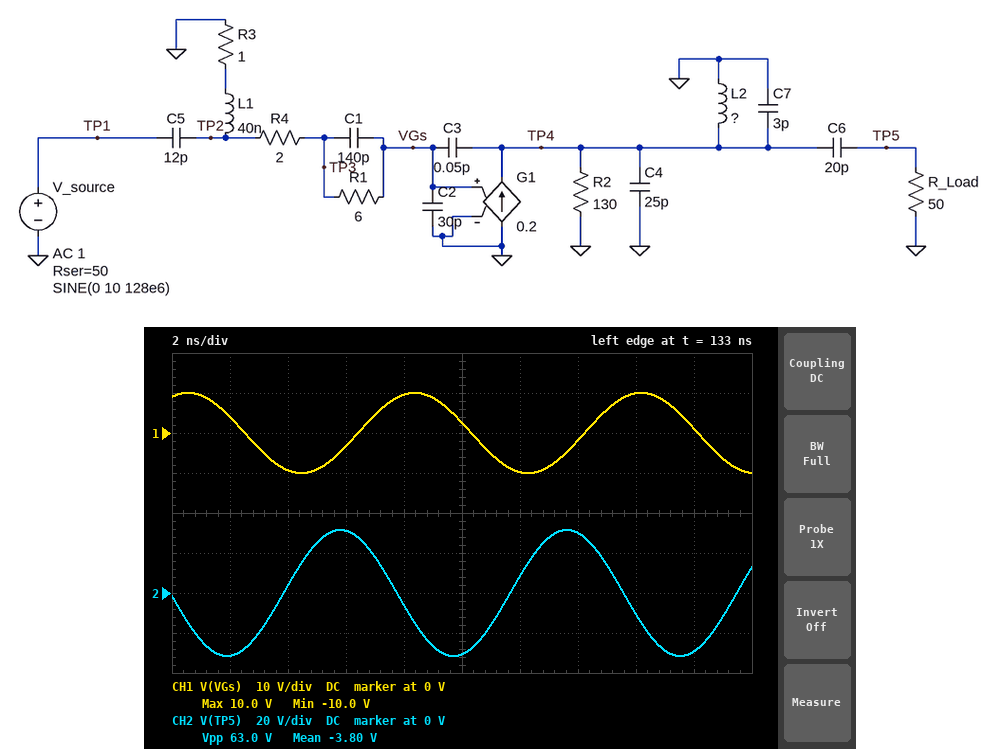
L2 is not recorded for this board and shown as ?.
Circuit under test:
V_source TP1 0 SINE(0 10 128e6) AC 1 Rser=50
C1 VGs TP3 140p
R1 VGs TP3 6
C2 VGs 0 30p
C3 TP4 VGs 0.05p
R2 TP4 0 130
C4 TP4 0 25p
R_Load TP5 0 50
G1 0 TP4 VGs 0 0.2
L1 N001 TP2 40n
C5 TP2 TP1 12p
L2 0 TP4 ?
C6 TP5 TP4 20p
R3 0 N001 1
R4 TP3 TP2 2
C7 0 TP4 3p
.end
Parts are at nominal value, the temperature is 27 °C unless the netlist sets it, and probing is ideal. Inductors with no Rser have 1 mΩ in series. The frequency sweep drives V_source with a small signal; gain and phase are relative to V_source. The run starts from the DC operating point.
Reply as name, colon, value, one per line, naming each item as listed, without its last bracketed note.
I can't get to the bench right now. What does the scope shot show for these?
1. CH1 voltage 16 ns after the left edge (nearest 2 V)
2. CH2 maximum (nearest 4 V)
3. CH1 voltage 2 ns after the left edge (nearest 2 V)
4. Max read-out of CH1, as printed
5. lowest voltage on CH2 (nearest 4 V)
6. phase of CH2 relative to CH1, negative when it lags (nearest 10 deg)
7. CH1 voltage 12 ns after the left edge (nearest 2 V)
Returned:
CH1 voltage 16 ns after the left edge: 10 V
CH2 maximum: 32 V
CH1 voltage 2 ns after the left edge: 4 V
Max read-out of CH1, as printed: 10.0 V
lowest voltage on CH2: -32 V
phase of CH2 relative to CH1, negative when it lags: 120 deg
CH1 voltage 12 ns after the left edge: -10 V
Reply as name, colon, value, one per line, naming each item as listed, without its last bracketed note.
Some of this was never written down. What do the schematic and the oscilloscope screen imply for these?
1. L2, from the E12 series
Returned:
L2, from the E12 series: 18 nH
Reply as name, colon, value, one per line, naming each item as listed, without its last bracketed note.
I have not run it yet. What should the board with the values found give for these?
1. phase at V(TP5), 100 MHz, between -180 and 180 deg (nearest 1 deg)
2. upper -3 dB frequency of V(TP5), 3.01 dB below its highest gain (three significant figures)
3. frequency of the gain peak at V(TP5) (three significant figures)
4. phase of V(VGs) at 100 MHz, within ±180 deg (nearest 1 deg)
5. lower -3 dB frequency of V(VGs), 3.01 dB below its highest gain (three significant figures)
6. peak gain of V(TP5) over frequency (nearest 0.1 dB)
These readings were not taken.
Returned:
phase at V(TP5), 100 MHz, between -180 and 180 deg: -94 deg
upper -3 dB frequency of V(TP5), 3.01 dB below its highest gain: 222 MHz
frequency of the gain peak at V(TP5): 172 MHz
phase of V(VGs) at 100 MHz, within ±180 deg: 130 deg
lower -3 dB frequency of V(VGs), 3.01 dB below its highest gain: 114 MHz
peak gain of V(TP5) over frequency: 11.3 dB
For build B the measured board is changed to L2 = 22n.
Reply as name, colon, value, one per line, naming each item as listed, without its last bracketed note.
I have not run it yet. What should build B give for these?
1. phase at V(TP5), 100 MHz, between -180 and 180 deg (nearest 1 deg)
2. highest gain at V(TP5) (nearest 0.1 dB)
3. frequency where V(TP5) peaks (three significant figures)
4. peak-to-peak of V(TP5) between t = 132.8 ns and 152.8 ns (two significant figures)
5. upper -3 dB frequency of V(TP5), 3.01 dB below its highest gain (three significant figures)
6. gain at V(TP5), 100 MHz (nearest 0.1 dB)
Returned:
phase at V(TP5), 100 MHz, between -180 and 180 deg: -98 deg
highest gain at V(TP5): 14.0 dB
frequency where V(TP5) peaks: 142 MHz
peak-to-peak of V(TP5) between t = 132.8 ns and 152.8 ns: 87 V
upper -3 dB frequency of V(TP5), 3.01 dB below its highest gain: 187 MHz
gain at V(TP5), 100 MHz: -0.9 dB
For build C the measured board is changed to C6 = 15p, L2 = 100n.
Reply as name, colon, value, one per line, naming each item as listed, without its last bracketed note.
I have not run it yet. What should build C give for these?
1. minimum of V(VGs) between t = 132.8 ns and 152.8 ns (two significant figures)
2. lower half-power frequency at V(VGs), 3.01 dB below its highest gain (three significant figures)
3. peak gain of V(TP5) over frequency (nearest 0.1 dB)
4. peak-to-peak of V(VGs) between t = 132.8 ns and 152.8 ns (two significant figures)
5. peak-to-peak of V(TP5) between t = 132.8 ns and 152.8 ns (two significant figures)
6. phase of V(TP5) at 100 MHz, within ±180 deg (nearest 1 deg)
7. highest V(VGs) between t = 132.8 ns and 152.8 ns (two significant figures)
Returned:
minimum of V(VGs) between t = 132.8 ns and 152.8 ns: -11 V
lower half-power frequency at V(VGs), 3.01 dB below its highest gain: 115 MHz
peak gain of V(TP5) over frequency: 13.6 dB
peak-to-peak of V(VGs) between t = 132.8 ns and 152.8 ns: 21 V
peak-to-peak of V(TP5) between t = 132.8 ns and 152.8 ns: 95 V
phase of V(TP5) at 100 MHz, within ±180 deg: 157 deg
highest V(VGs) between t = 132.8 ns and 152.8 ns: 11 V
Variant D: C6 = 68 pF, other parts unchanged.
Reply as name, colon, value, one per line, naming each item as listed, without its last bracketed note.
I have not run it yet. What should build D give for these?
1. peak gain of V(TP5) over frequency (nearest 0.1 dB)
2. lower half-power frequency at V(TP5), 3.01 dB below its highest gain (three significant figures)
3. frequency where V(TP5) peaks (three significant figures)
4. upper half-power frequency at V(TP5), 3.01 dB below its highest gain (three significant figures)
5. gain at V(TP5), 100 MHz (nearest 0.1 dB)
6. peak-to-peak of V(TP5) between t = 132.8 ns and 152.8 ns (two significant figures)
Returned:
peak gain of V(TP5) over frequency: 12.5 dB
lower half-power frequency at V(TP5), 3.01 dB below its highest gain: 119 MHz
frequency where V(TP5) peaks: 135 MHz
upper half-power frequency at V(TP5), 3.01 dB below its highest gain: 200 MHz
gain at V(TP5), 100 MHz: 0.7 dB
peak-to-peak of V(TP5) between t = 132.8 ns and 152.8 ns: 80 V
